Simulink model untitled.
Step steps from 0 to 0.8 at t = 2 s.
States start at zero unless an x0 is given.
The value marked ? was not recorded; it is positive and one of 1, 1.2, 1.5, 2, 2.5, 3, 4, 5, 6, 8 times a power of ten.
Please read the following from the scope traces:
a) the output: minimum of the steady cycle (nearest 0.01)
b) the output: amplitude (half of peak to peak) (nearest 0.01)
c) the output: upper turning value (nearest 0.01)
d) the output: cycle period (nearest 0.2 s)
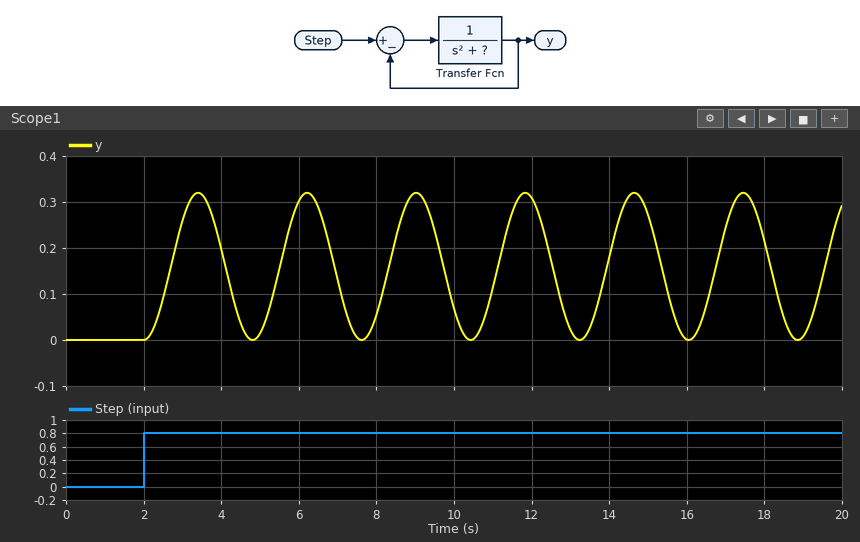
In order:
0.00
0.16
0.32
2.8 s
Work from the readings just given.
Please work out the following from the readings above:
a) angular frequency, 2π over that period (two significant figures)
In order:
2.2 rad/s
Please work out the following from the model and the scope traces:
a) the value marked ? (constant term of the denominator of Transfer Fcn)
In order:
4
